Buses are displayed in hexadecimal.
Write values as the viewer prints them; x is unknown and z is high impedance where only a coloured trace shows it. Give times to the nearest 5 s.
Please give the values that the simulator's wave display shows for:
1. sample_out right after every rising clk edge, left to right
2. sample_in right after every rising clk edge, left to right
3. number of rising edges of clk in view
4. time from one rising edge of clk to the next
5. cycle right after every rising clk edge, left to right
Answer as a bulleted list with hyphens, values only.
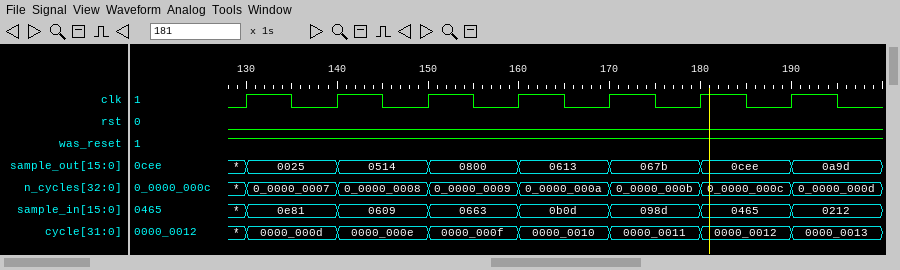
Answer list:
- 0025, 0514, 0800, 0613, 067b, 0cee, 0a9d
- 0e81, 0609, 0663, 0b0d, 098d, 0465, 0212
- 7
- 10 s
- 0000_000d, 0000_000e, 0000_000f, 0000_0010, 0000_0011, 0000_0012, 0000_0013
